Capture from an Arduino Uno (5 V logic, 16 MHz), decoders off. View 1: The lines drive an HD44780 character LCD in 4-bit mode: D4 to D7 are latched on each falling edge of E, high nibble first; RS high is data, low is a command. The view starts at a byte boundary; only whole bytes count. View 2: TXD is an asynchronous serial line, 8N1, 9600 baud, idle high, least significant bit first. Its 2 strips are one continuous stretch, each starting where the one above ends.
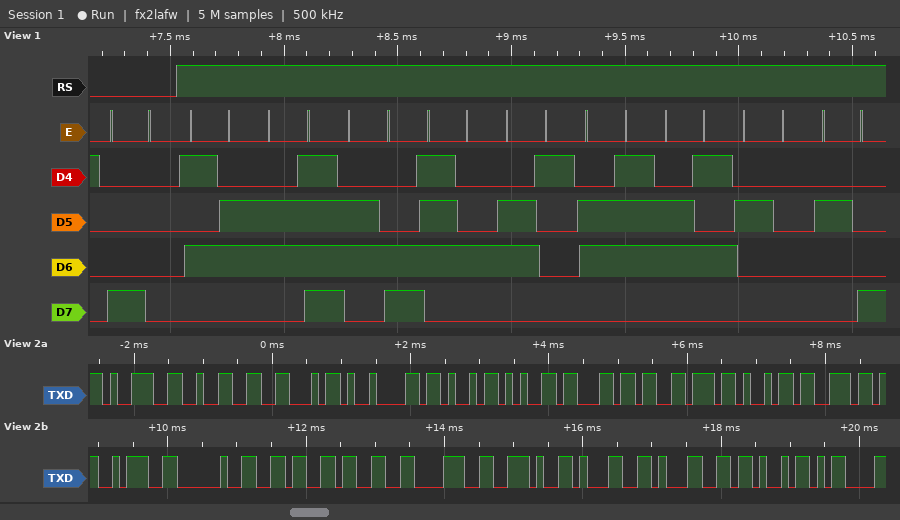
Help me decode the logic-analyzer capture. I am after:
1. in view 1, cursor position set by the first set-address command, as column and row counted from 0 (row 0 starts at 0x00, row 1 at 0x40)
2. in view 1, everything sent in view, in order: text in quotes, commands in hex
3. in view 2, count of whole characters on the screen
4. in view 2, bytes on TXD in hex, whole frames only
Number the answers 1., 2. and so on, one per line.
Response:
1. column 0, row 0
2. 0x80 "Voltage ("
3. 20
4. 0x39 0x32 0x46 0x09 0x4B 0x65 0x6C 0x76 0x69 0x6E 0x3A 0x20 0x36 0x33 0x38 0x2E 0x31 0x31 0x4B 0x0D
